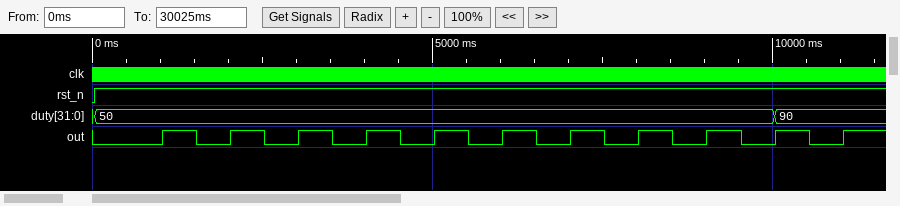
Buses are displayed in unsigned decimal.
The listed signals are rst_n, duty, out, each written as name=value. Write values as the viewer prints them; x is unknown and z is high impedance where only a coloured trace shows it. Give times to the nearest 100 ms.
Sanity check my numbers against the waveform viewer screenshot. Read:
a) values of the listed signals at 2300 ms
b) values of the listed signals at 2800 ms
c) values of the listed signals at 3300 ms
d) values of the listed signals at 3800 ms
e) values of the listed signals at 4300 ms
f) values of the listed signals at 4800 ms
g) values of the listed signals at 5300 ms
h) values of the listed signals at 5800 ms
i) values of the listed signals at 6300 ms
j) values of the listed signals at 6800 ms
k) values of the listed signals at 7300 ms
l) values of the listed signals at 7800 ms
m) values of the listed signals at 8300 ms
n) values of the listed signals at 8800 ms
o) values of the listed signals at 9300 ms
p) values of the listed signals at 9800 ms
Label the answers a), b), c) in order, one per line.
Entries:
a) rst_n=1, duty=50, out=1
b) rst_n=1, duty=50, out=0
c) rst_n=1, duty=50, out=1
d) rst_n=1, duty=50, out=0
e) rst_n=1, duty=50, out=1
f) rst_n=1, duty=50, out=0
g) rst_n=1, duty=50, out=1
h) rst_n=1, duty=50, out=0
i) rst_n=1, duty=50, out=1
j) rst_n=1, duty=50, out=0
k) rst_n=1, duty=50, out=1
l) rst_n=1, duty=50, out=0
m) rst_n=1, duty=50, out=1
n) rst_n=1, duty=50, out=0
o) rst_n=1, duty=50, out=1
p) rst_n=1, duty=50, out=0
